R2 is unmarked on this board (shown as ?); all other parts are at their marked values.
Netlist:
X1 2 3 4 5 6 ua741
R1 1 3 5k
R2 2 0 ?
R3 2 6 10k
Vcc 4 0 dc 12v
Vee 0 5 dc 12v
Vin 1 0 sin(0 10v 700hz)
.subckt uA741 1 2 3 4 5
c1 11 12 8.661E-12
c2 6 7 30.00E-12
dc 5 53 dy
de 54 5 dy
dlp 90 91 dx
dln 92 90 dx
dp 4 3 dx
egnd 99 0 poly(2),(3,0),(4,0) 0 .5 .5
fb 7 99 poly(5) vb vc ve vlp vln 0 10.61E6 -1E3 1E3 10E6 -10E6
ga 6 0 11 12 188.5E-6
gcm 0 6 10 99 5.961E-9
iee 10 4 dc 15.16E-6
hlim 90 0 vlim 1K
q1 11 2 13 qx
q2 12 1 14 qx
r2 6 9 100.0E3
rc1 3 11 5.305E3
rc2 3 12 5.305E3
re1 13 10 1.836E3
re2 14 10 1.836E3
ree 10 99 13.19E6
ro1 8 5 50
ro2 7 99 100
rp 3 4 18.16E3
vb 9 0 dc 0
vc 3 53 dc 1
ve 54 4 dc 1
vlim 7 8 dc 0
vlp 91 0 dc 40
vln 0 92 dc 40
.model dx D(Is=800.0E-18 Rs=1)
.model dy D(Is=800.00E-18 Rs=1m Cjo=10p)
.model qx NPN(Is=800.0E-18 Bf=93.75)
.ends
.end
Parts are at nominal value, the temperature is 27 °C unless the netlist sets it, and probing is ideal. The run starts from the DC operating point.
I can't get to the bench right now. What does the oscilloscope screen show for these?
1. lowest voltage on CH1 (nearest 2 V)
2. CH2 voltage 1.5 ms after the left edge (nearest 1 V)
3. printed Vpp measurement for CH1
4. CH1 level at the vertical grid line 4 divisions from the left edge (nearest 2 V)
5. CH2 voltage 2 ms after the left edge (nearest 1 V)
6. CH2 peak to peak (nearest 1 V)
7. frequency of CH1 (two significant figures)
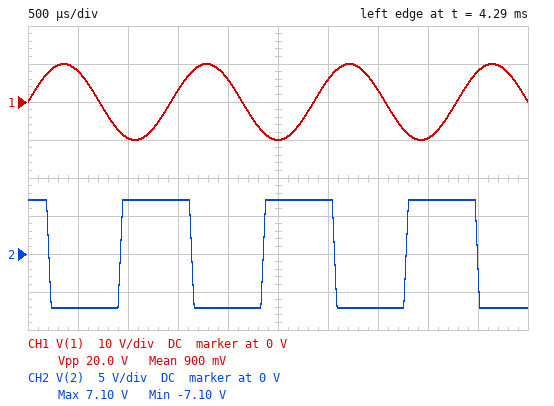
-10 V
7 V
20.0 V
6 V
-7 V
14 V
700 Hz
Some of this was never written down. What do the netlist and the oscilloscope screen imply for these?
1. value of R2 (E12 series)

15 kΩ
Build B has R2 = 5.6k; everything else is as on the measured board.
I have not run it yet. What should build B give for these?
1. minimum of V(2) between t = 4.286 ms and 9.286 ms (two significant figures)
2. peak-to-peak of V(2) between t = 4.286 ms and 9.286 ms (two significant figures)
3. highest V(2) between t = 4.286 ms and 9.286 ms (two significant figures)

-4.2 V
8.5 V
4.2 V
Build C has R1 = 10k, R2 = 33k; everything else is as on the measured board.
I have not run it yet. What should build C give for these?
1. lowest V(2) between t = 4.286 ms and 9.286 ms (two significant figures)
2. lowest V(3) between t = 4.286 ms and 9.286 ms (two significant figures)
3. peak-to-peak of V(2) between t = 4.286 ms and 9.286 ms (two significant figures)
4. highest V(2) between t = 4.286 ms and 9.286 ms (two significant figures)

-9.1 V
-10 V
18 V
9.1 V
